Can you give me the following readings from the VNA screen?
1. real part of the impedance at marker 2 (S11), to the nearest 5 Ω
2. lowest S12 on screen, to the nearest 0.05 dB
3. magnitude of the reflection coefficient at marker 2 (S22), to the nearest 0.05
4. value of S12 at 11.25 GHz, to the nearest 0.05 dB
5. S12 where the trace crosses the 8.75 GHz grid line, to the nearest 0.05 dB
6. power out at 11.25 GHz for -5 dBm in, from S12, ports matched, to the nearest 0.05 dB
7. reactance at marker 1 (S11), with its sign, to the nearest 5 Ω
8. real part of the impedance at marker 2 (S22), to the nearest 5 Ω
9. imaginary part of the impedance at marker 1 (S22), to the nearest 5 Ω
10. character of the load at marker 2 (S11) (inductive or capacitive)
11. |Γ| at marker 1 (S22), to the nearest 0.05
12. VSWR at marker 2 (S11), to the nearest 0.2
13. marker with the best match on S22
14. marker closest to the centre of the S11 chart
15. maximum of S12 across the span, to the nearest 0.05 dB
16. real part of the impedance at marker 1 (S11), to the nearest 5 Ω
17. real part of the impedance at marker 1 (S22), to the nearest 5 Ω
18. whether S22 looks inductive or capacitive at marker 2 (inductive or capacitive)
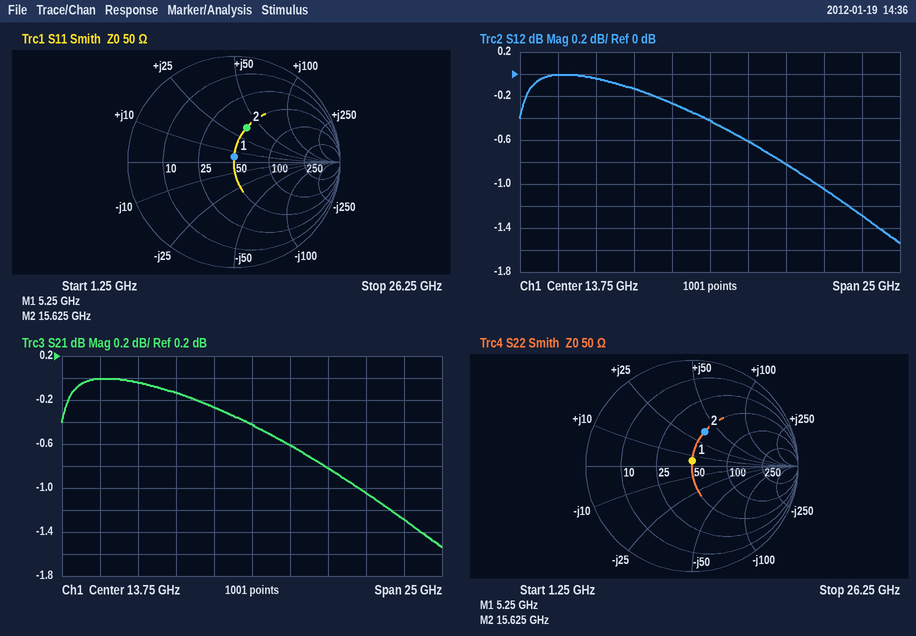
50 Ω
-1.55 dB
0.35
-0.25 dB
-0.15 dB
-5.25 dBm
+5 Ω
50 Ω
+5 Ω
inductive
0.05
2.0
marker 1
marker 1
0.00 dB
50 Ω
50 Ω
inductive
